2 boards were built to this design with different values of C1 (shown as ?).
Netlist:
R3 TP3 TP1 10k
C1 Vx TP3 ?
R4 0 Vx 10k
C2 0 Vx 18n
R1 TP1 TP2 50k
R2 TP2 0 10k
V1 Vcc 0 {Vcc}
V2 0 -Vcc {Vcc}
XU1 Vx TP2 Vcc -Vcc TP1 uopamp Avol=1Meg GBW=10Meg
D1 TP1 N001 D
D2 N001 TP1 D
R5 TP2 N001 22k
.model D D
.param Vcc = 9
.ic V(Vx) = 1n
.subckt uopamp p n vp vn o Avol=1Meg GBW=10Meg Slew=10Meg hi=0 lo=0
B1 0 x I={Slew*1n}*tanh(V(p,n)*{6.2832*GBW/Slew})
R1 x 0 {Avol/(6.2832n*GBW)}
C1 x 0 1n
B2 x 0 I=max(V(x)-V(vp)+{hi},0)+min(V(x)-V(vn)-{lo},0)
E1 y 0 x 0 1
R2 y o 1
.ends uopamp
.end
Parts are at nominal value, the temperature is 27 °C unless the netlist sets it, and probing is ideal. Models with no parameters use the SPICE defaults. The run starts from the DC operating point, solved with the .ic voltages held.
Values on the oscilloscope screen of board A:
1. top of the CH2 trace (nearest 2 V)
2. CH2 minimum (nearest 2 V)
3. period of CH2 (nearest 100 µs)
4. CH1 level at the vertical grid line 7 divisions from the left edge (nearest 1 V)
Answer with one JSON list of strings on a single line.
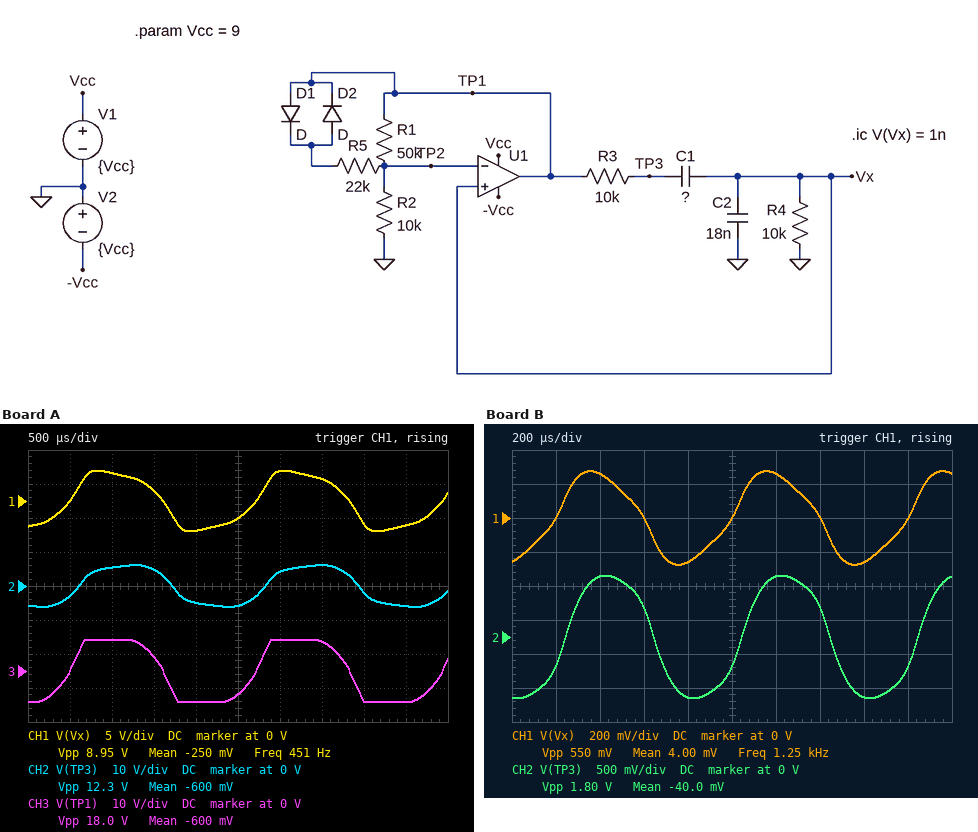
["6 V", "-6 V", "2.2 ms", "3 V"]
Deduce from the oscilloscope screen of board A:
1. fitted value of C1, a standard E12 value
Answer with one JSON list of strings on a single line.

["56 nF"]
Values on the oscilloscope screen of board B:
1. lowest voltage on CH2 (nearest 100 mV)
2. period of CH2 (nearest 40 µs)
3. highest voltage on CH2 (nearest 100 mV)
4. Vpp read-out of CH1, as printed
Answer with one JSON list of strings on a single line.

["-900 mV", "800 µs", "900 mV", "550 mV"]
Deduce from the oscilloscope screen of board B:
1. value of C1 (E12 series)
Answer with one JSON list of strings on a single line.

["8.2 nF"]
